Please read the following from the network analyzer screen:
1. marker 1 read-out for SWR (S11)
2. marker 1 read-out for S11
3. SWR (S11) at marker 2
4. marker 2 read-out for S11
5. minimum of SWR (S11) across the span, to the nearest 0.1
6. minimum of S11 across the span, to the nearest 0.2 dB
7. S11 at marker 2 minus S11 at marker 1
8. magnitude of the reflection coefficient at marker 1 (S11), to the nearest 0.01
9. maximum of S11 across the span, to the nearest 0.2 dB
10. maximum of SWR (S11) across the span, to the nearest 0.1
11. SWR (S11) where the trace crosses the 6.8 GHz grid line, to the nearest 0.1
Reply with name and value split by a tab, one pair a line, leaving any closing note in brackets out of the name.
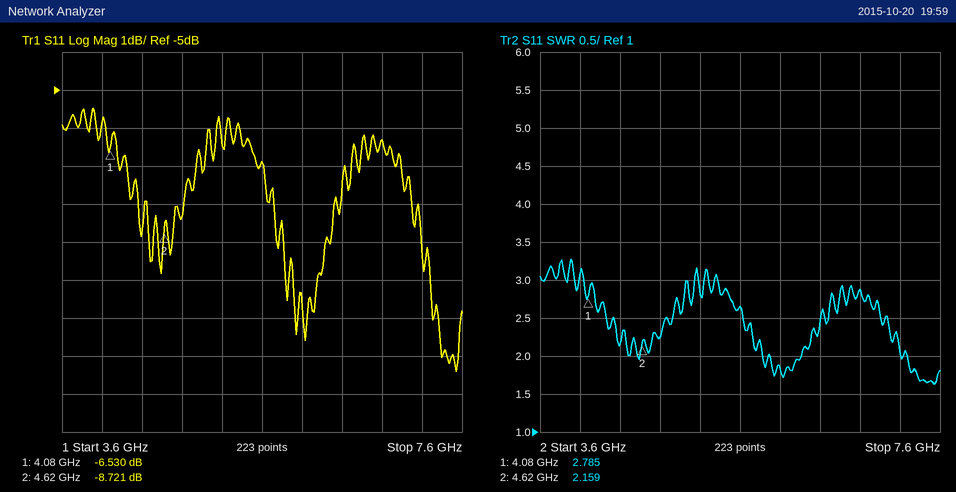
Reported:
marker 1 read-out for SWR	2.785
marker 1 read-out for S11	-6.530 dB
SWR (S11) at marker 2	2.159
marker 2 read-out for S11	-8.721 dB
minimum of SWR (S11) across the span, to the nearest 0.1	1.6
minimum of S11 across the span, to the nearest 0.2 dB	-12.4 dB
S11 at marker 2 minus S11 at marker 1	-2.191 dB
magnitude of the reflection coefficient at marker 1 (S11), to the nearest 0.01	0.47
maximum of S11 across the span, to the nearest 0.2 dB	-5.4 dB
maximum of SWR (S11) across the span, to the nearest 0.1	3.3
SWR (S11) where the trace crosses the 6.8 GHz grid line, to the nearest 0.1	2.9
